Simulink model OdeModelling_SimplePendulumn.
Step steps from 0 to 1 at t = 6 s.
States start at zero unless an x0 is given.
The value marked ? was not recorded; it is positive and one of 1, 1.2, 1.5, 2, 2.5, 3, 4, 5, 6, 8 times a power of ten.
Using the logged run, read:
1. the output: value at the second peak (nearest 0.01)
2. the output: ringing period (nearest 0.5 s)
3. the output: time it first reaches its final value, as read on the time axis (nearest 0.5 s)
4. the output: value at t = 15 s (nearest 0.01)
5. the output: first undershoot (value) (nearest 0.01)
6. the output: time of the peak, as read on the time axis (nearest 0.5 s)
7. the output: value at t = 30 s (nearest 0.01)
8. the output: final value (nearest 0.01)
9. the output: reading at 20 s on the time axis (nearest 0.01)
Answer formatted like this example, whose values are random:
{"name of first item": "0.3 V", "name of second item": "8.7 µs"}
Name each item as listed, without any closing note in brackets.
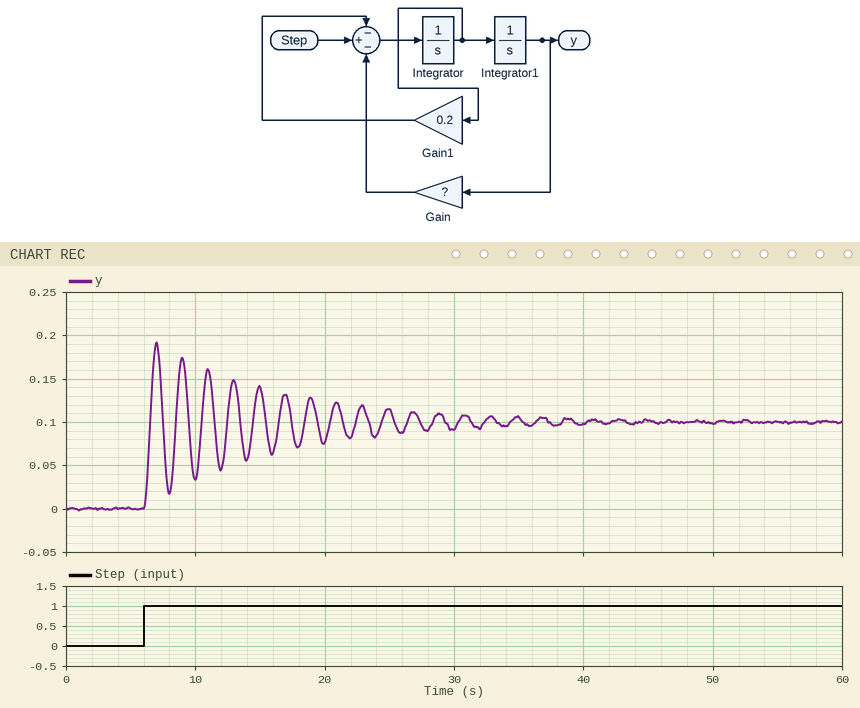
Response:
{"the output: value at the second peak": "0.17", "the output: ringing period": "2.0 s", "the output: time it first reaches its final value, as read on the time axis": "6.5 s", "the output: value at t = 15 s": "0.14", "the output: first undershoot (value)": "0.02", "the output: time of the peak, as read on the time axis": "7.0 s", "the output: value at t = 30 s": "0.09", "the output: final value": "0.10", "the output: reading at 20 s on the time axis": "0.08"}
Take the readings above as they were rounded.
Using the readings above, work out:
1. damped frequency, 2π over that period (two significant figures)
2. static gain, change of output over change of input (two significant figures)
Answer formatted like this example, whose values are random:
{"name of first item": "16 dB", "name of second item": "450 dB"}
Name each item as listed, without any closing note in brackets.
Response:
{"damped frequency, 2π over that period": "3.1 rad/s", "static gain, change of output over change of input": "0.10"}
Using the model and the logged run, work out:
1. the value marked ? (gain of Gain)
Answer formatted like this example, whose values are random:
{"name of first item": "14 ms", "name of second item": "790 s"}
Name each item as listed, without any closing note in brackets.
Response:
{"the value marked ?": "10"}
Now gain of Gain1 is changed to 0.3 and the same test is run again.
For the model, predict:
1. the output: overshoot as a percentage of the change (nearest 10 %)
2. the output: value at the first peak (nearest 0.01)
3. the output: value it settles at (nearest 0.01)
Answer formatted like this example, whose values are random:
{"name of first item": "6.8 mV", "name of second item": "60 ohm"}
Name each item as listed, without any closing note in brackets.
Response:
{"the output: overshoot as a percentage of the change": "90 %", "the output: value at the first peak": "0.19", "the output: value it settles at": "0.10"}
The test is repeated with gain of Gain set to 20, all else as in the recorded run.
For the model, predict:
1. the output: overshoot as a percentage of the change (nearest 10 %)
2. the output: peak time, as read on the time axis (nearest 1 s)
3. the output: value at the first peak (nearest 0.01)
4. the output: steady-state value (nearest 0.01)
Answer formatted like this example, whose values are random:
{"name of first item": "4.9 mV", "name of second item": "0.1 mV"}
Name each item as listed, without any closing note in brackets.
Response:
{"the output: overshoot as a percentage of the change": "90 %", "the output: peak time, as read on the time axis": "7 s", "the output: value at the first peak": "0.10", "the output: steady-state value": "0.05"}
